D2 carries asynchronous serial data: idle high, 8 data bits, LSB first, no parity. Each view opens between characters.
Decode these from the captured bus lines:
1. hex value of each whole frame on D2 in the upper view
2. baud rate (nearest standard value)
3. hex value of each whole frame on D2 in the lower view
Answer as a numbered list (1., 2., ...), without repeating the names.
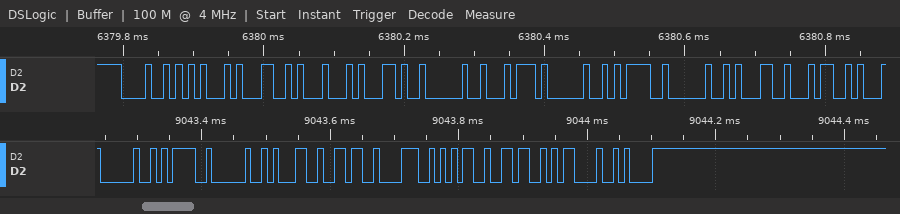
1. 48, 45, 4C, 44, 2C, 20, 74, 20, 3D, 20, 31, 34
2. 115200 baud
3. 20, 3D, 20, 31, 36, 38, 35, 36, 0D, 0A
